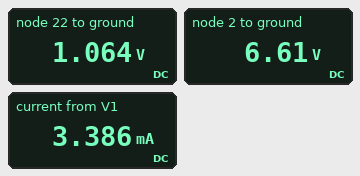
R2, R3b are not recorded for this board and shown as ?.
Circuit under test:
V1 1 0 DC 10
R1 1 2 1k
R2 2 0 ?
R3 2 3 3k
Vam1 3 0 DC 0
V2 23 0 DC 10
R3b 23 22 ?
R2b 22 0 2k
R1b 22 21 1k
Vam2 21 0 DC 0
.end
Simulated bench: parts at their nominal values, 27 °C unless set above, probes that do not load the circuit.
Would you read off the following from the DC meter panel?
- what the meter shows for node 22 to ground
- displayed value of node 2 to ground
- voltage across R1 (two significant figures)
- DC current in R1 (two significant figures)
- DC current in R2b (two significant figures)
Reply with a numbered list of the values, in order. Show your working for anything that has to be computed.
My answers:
1. 1.064 V
2. 6.61 V
3. 10 V - 6.61 V = 3.4 V
4. (10 V - 6.61 V) / 1 kΩ = 3.4 mA
5. (1.064 V) / 2 kΩ = 530 µA
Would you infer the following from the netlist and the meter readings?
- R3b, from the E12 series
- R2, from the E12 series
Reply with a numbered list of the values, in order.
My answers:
1. 5.6 kΩ
2. 5.6 kΩ
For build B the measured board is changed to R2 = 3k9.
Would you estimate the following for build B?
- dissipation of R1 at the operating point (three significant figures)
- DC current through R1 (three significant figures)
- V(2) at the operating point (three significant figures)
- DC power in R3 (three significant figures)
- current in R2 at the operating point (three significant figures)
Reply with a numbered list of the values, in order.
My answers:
1. 13.8 mW
2. 3.71 mA
3. 6.29 V
4. 13.2 mW
5. 1.61 mA
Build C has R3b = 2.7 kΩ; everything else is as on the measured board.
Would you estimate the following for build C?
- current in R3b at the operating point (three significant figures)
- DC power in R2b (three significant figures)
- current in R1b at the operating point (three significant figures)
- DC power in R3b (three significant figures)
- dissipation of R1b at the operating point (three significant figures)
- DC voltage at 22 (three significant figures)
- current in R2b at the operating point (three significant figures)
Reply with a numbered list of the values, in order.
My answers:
1. 2.97 mA
2. 1.96 mW
3. 1.98 mA
4. 23.8 mW
5. 3.92 mW
6. 1.98 V
7. 990 µA
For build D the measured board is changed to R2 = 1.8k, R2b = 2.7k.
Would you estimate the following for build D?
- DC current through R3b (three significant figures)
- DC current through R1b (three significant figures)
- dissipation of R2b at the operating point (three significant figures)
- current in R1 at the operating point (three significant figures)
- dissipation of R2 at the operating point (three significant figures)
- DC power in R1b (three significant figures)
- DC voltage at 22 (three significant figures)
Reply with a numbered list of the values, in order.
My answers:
1. 1.58 mA
2. 1.15 mA
3. 492 µW
4. 4.71 mA
5. 15.6 mW
6. 1.33 mW
7. 1.15 V
